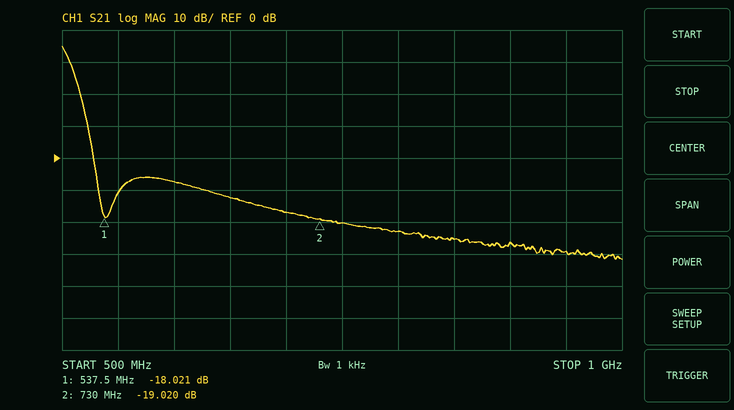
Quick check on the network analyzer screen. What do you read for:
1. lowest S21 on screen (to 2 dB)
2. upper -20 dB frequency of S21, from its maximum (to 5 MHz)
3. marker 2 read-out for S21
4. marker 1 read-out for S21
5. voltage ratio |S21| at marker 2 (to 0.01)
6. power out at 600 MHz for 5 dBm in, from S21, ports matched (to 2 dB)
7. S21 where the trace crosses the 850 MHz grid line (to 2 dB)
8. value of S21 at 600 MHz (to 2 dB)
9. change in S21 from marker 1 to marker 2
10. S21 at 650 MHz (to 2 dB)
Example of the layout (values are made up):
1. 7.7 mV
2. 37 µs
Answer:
1. -32 dB
2. 520 MHz
3. -19.020 dB
4. -18.021 dB
5. 0.11
6. -2 dBm
7. -26 dB
8. -8 dB
9. -0.999 dB
10. -12 dB
